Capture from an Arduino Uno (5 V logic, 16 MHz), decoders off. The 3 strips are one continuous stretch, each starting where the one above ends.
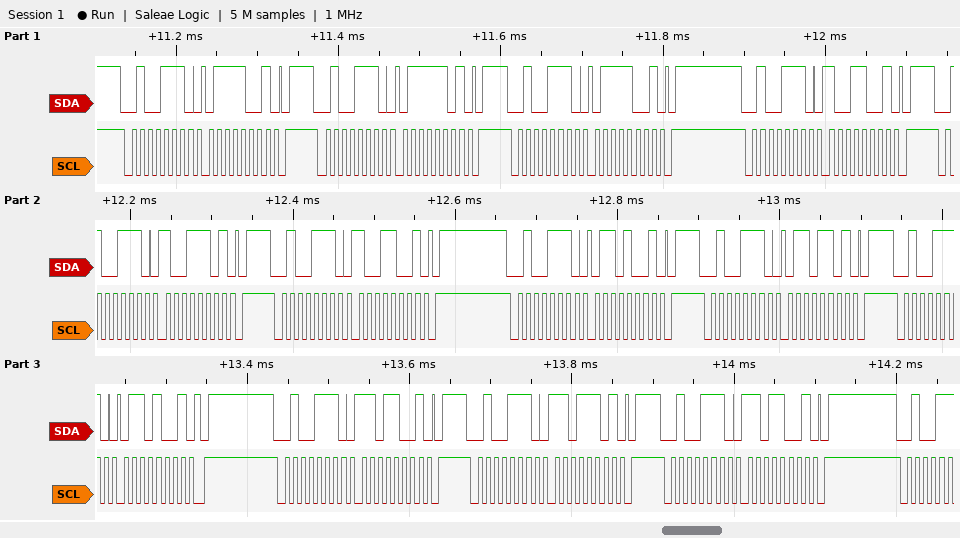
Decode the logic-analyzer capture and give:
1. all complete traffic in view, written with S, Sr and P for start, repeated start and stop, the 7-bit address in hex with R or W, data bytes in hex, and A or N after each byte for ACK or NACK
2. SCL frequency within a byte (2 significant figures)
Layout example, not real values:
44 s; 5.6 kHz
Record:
S 27W A 79 A P S 27W A 7D A P S 27W A 79 A P S 27W A 99 A P S 27W A 9D A P S 27W A 99 A P S 27W A 69 A P S 27W A 6D A P S 27W A 69 A P S 27W A D9 A P S 27W A DD A P S 27W A D9 A P; 100 kHz
